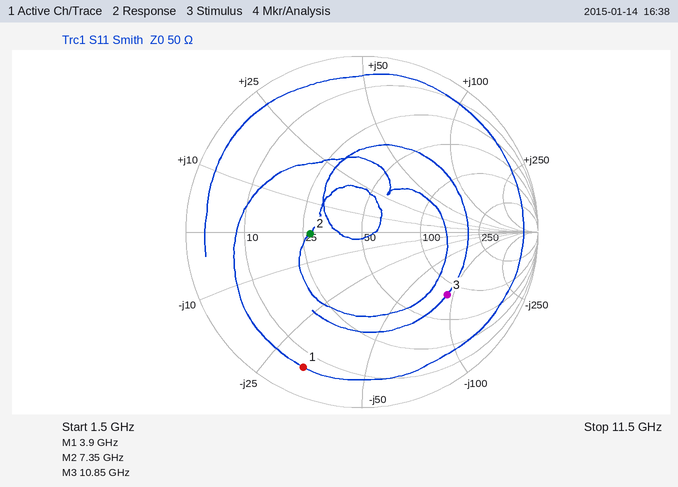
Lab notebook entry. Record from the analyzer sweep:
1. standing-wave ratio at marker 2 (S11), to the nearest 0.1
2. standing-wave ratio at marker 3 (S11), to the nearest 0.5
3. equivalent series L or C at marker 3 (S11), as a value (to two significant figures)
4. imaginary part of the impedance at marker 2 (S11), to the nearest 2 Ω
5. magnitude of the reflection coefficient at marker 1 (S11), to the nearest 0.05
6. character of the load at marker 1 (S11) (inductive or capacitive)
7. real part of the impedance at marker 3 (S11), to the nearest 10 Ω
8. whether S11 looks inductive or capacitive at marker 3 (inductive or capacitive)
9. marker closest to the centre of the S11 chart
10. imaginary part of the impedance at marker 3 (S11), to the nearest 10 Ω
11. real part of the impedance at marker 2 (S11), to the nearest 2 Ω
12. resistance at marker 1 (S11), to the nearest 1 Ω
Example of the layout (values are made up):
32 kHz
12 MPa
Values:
1.8
4.0
160 fF
0 Ω
0.85
capacitive
80 Ω
capacitive
marker 2
-90 Ω
28 Ω
6 Ω
